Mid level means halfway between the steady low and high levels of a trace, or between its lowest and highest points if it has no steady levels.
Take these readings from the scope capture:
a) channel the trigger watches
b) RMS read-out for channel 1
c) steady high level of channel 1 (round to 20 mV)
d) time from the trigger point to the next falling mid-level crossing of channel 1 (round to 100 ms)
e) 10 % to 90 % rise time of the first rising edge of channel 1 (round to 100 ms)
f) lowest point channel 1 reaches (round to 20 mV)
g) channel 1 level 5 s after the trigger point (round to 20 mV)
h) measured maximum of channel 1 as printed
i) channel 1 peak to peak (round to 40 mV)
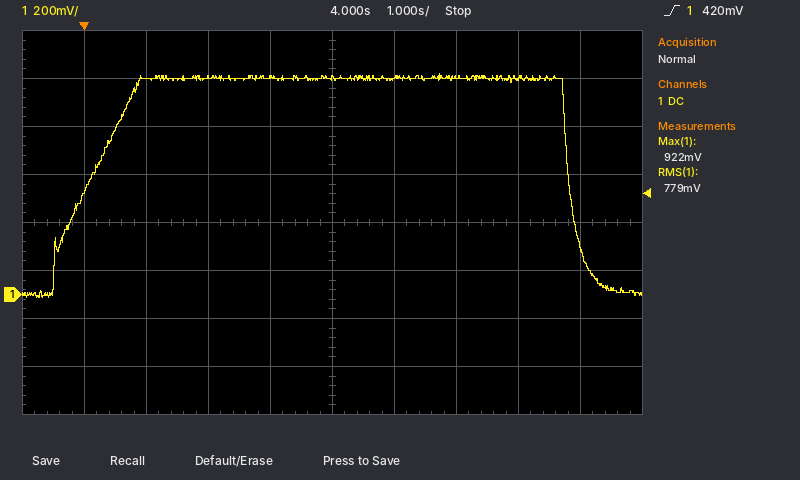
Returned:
channel 1
779 mV
900 mV
7.8 s
1.2 s
-20 mV
900 mV
922 mV
920 mV
